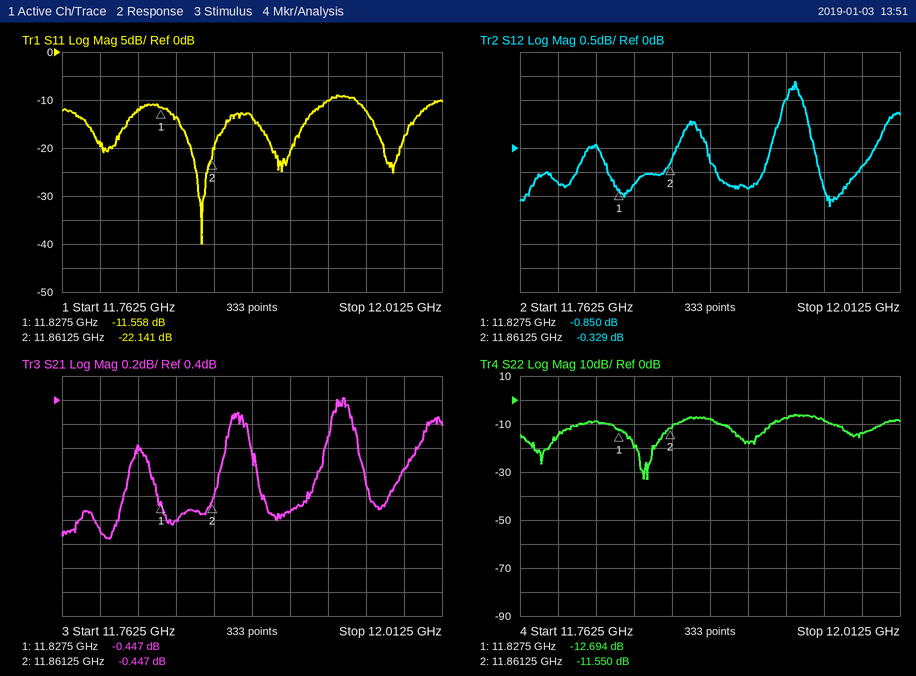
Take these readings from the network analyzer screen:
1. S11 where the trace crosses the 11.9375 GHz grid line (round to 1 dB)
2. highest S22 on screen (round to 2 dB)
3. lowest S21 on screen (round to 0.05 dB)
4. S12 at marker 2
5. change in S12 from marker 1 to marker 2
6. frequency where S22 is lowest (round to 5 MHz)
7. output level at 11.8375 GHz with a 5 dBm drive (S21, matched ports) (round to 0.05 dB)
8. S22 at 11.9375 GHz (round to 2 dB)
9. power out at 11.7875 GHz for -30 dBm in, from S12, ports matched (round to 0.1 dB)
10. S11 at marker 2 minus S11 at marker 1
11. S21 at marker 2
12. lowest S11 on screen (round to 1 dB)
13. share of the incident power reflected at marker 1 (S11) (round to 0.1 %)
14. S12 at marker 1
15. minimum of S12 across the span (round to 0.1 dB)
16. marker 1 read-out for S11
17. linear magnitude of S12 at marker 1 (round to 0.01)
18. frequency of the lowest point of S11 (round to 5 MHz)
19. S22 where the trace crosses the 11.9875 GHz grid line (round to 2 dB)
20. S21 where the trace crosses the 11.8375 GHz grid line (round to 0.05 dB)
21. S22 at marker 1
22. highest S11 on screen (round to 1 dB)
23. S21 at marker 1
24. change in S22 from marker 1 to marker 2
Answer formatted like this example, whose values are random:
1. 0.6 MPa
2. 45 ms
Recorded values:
1. -10 dB
2. -6 dB
3. -0.75 dB
4. -0.329 dB
5. 0.521 dB
6. 11.845 GHz
7. 4.40 dBm
8. -8 dB
9. -30.7 dBm
10. -10.583 dB
11. -0.447 dB
12. -40 dB
13. 7.0 %
14. -0.850 dB
15. -1.2 dB
16. -11.558 dB
17. 0.91
18. 11.855 GHz
19. -14 dB
20. -0.60 dB
21. -12.694 dB
22. -9 dB
23. -0.447 dB
24. 1.144 dB
